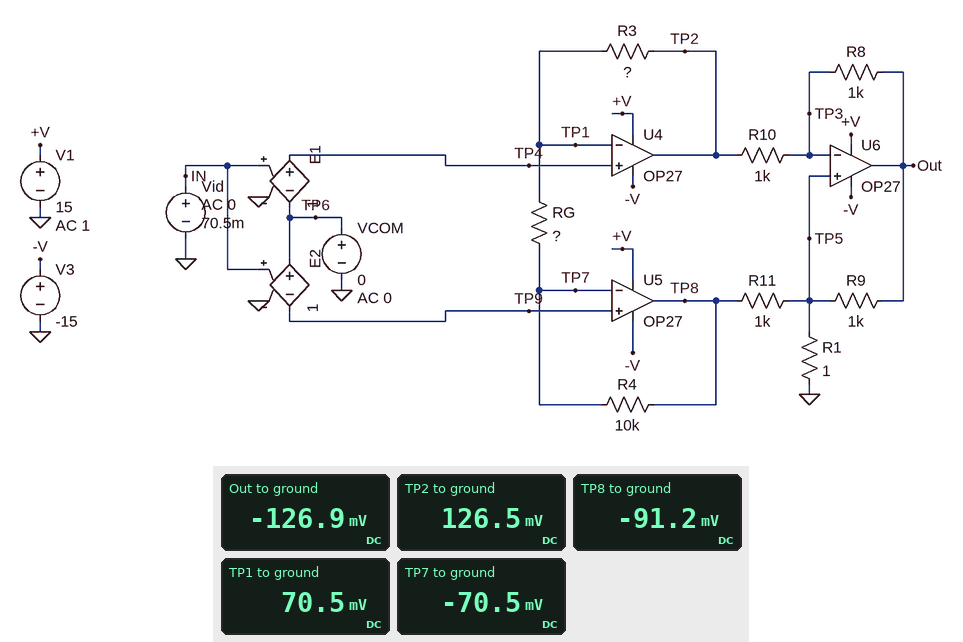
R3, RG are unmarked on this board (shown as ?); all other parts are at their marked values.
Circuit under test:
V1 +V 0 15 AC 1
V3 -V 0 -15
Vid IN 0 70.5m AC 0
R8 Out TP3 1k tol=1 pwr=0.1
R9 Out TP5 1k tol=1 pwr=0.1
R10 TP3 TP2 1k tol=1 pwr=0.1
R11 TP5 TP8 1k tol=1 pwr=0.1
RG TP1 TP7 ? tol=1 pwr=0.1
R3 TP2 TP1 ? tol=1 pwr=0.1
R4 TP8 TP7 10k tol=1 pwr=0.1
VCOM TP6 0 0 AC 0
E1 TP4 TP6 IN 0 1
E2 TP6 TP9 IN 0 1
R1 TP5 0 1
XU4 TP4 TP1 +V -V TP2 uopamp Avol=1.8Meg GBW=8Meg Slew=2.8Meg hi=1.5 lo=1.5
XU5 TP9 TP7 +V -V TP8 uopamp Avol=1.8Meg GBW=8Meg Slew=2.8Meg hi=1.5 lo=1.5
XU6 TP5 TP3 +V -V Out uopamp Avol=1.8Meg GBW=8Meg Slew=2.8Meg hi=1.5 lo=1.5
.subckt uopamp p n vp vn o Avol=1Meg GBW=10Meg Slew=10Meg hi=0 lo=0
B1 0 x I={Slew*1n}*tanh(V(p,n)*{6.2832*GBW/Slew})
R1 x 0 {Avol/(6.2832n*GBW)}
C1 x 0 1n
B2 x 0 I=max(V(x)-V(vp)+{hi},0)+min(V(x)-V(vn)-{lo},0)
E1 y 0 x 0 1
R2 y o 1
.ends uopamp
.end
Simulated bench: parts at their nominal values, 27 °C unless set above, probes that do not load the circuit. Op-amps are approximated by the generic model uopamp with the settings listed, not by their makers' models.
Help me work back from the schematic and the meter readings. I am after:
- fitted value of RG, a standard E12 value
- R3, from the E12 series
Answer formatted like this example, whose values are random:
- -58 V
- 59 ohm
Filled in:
- 68 kΩ
- 27 kΩ
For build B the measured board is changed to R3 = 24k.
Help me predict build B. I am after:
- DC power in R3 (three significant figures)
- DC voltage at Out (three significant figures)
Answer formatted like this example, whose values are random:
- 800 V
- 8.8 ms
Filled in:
- 103 nW
- -121 mV
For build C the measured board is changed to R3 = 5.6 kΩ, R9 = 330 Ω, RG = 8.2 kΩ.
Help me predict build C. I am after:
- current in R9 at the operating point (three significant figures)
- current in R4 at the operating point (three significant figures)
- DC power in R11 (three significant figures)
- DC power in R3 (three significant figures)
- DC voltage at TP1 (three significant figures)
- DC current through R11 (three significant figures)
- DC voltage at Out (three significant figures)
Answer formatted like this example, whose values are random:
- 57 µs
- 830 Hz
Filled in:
- 508 µA
- 17.2 µA
- 58.4 µW
- 1.66 µW
- 70.5 mV
- 242 µA
- -168 mV
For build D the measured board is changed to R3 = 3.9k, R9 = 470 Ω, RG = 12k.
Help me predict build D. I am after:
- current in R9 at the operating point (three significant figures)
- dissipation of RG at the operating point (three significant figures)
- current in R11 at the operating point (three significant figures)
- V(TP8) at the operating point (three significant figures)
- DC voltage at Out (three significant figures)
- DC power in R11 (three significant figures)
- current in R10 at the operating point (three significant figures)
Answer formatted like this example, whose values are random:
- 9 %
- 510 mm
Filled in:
- 248 µA
- 1.66 µW
- 188 µA
- -188 mV
- -117 mV
- 35.2 µW
- 117 µA
